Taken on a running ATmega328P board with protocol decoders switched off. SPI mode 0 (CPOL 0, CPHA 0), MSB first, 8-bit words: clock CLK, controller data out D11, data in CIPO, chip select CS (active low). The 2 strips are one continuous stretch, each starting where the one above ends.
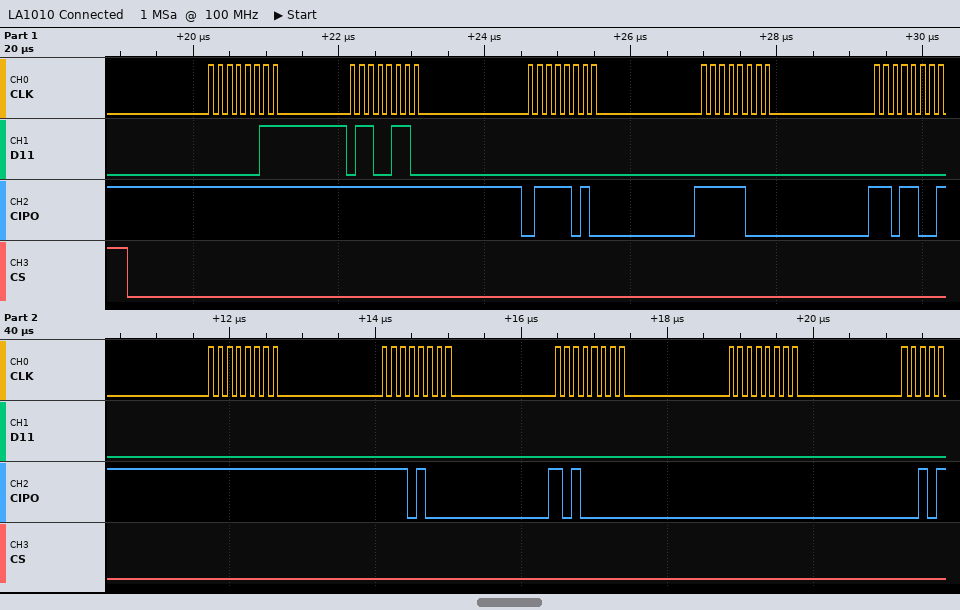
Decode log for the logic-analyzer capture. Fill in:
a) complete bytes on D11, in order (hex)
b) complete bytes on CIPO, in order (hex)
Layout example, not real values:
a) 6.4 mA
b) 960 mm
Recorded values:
a) 03 66 00 00 00 00 00 00 00
b) FF FF 7A F8 D9 FF E8 A0 00
